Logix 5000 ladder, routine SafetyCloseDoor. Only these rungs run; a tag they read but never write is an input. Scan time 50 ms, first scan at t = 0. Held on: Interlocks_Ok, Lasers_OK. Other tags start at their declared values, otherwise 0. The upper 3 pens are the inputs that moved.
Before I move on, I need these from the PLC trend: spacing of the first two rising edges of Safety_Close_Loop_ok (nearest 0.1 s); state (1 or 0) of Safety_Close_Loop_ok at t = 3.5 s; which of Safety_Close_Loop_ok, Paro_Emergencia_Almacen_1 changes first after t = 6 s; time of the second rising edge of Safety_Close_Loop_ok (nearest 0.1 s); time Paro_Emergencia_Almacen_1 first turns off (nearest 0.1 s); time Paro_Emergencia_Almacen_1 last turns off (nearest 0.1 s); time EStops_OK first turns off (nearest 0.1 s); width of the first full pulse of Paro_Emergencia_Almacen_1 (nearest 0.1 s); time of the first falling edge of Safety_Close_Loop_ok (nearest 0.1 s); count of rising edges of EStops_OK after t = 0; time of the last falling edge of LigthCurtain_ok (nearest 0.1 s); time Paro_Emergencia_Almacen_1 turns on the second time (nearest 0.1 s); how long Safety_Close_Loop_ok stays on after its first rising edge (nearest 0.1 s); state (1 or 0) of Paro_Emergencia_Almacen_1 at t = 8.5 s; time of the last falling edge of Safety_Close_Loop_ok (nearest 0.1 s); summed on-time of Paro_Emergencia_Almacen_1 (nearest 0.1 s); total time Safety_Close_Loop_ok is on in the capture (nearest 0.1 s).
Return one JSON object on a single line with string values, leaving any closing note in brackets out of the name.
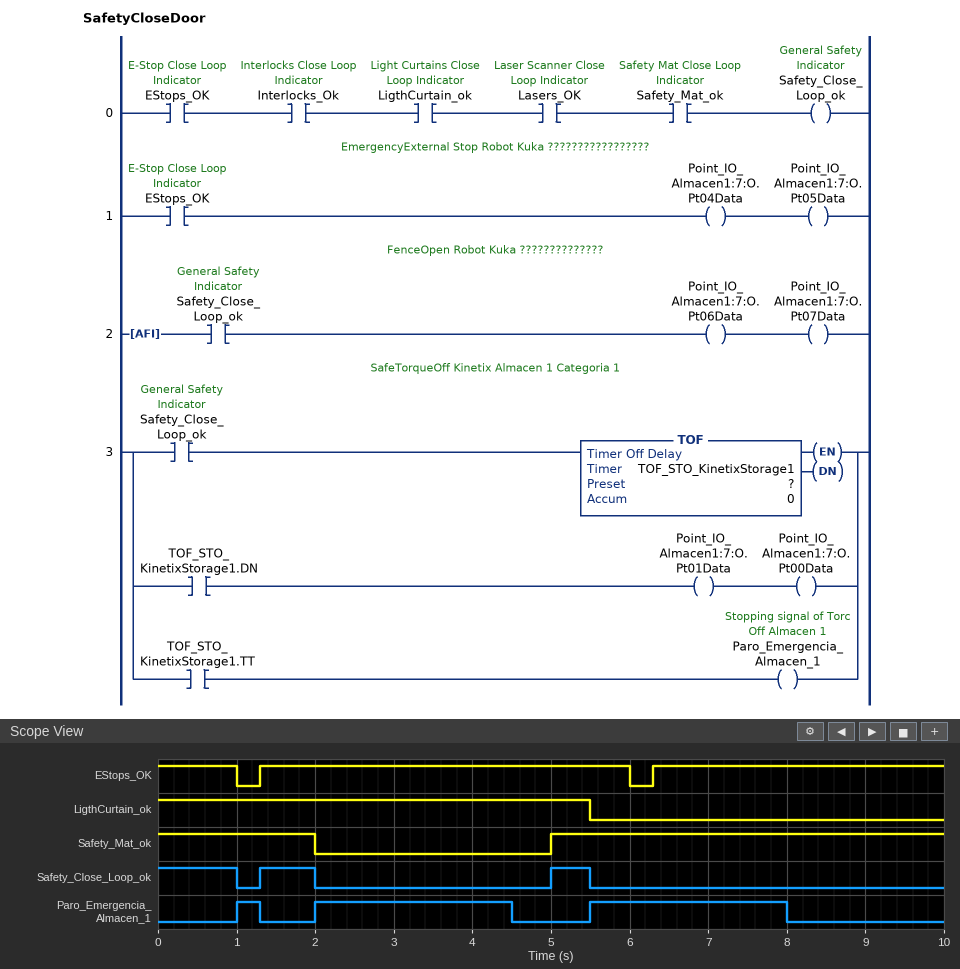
{"spacing of the first two rising edges of Safety_Close_Loop_ok": "3.7 s", "state (1 or 0) of Safety_Close_Loop_ok at t = 3.5 s": "0", "which of Safety_Close_Loop_ok, Paro_Emergencia_Almacen_1 changes first after t = 6 s": "Paro_Emergencia_Almacen_1", "time of the second rising edge of Safety_Close_Loop_ok": "5.0 s", "time Paro_Emergencia_Almacen_1 first turns off": "1.3 s", "time Paro_Emergencia_Almacen_1 last turns off": "8.0 s", "time EStops_OK first turns off": "1.0 s", "width of the first full pulse of Paro_Emergencia_Almacen_1": "0.3 s", "time of the first falling edge of Safety_Close_Loop_ok": "1.0 s", "count of rising edges of EStops_OK after t = 0": "2", "time of the last falling edge of LigthCurtain_ok": "5.5 s", "time Paro_Emergencia_Almacen_1 turns on the second time": "2.0 s", "how long Safety_Close_Loop_ok stays on after its first rising edge": "0.7 s", "state (1 or 0) of Paro_Emergencia_Almacen_1 at t = 8.5 s": "0", "time of the last falling edge of Safety_Close_Loop_ok": "5.5 s", "summed on-time of Paro_Emergencia_Almacen_1": "5.3 s", "total time Safety_Close_Loop_ok is on in the capture": "2.2 s"}
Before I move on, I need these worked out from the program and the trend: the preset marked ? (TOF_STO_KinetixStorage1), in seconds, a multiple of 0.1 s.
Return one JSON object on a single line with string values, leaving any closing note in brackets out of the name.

{"the preset marked ? (TOF_STO_KinetixStorage1), in seconds, a multiple of 0.1 s": "2.5 s"}
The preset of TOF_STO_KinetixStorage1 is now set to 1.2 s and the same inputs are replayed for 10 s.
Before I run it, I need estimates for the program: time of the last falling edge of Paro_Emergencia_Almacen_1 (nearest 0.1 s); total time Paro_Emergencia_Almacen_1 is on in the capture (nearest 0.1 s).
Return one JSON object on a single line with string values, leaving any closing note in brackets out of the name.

{"time of the last falling edge of Paro_Emergencia_Almacen_1": "6.7 s", "total time Paro_Emergencia_Almacen_1 is on in the capture": "2.7 s"}
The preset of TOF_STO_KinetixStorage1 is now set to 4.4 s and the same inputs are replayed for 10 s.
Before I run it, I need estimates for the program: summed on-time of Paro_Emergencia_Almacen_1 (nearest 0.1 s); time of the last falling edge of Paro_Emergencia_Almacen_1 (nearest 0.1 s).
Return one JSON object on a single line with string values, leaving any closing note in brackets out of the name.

{"summed on-time of Paro_Emergencia_Almacen_1": "7.7 s", "time of the last falling edge of Paro_Emergencia_Almacen_1": "9.9 s"}
